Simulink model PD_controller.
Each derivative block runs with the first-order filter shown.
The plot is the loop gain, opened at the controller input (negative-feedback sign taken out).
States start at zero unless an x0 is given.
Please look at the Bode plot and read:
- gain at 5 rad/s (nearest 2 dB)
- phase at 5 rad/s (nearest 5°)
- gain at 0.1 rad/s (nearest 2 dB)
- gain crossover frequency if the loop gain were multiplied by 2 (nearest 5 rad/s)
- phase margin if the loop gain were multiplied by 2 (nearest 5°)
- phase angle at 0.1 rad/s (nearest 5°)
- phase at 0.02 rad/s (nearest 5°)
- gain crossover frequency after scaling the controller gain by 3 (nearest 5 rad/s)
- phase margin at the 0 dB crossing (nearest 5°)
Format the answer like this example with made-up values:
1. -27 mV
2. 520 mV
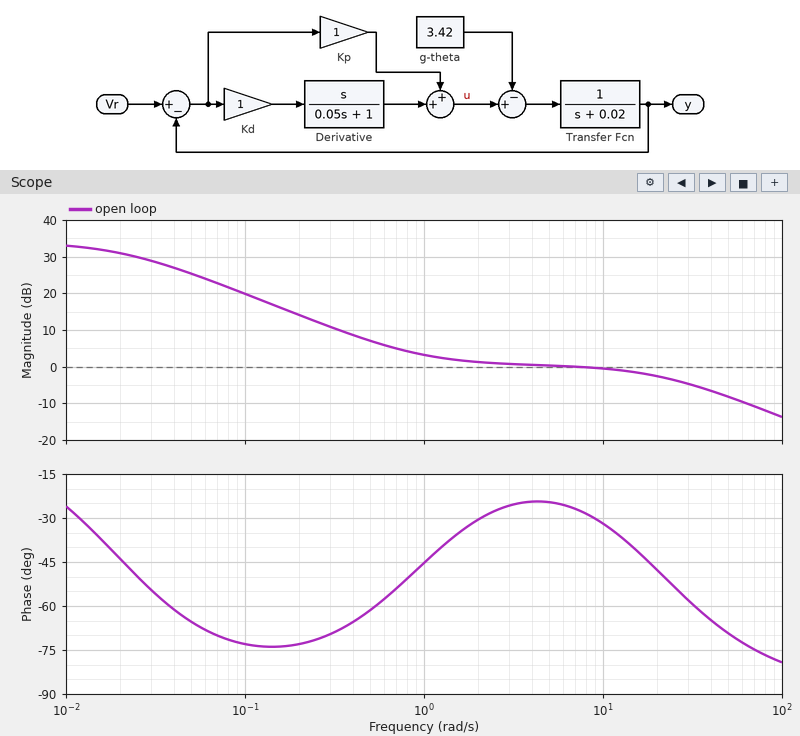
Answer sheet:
1. 0 dB
2. -25°
3. 20 dB
4. 35 rad/s
5. 115°
6. -75°
7. -45°
8. 60 rad/s
9. 155°
